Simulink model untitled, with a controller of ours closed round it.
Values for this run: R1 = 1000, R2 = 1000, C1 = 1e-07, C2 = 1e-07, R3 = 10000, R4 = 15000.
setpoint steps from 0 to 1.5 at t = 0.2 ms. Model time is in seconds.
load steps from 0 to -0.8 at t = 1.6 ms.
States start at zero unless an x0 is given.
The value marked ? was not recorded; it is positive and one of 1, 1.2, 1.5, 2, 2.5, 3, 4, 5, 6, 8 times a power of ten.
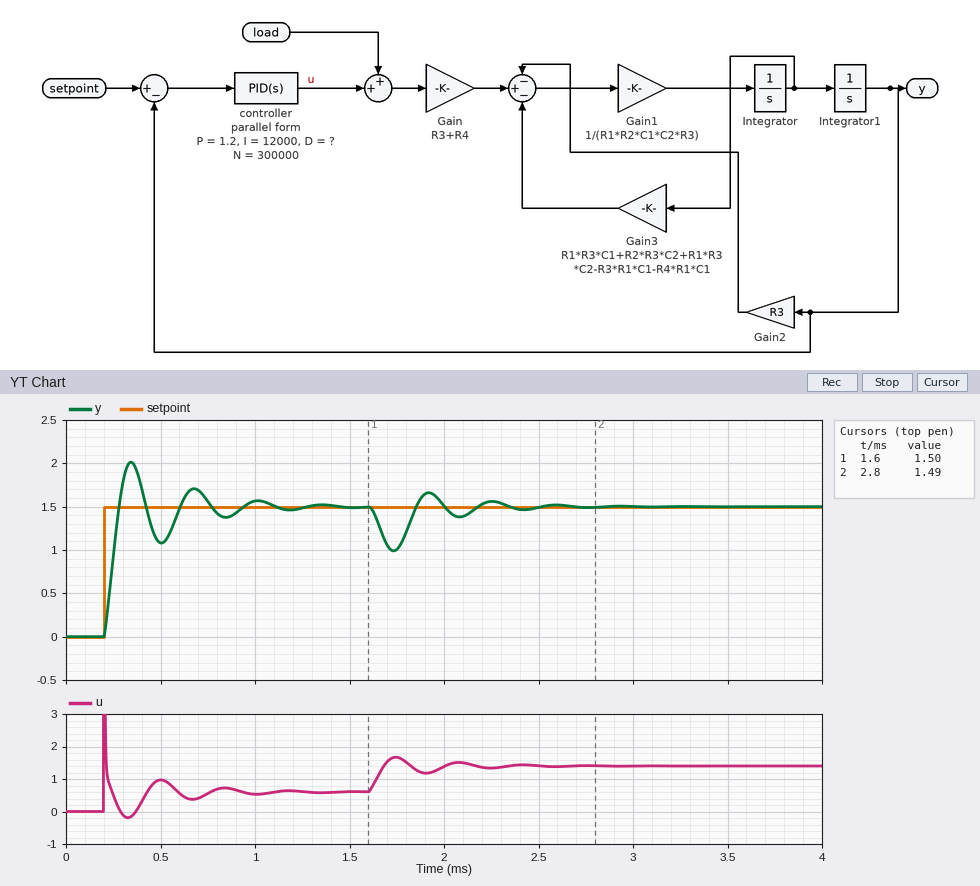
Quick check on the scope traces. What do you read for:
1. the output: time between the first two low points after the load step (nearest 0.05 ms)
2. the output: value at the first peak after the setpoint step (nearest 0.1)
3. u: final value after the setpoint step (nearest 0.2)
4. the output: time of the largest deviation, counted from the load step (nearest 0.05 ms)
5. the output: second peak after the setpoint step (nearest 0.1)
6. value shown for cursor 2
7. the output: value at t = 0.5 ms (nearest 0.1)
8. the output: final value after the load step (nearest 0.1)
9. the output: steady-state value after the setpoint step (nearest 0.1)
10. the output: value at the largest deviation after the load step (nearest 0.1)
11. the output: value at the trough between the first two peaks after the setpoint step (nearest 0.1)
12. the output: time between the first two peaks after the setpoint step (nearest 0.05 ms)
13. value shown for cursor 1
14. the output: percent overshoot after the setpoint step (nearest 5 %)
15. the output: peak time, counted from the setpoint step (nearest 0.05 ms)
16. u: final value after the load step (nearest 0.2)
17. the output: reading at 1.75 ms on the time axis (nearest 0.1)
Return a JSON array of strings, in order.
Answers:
["0.35 ms", "2.0", "0.6", "0.15 ms", "1.7", "1.49", "1.1", "1.5", "1.5", "1.0", "1.1", "0.35 ms", "1.50", "35 %", "0.15 ms", "1.4", "1.0"]
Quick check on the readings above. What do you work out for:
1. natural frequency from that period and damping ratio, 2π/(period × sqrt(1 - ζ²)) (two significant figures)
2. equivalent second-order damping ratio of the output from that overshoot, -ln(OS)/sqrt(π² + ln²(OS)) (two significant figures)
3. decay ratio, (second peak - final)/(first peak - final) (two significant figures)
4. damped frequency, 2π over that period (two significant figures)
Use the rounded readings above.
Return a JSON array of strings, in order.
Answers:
["19 rad/ms", "0.32", "0.40", "18 rad/ms"]
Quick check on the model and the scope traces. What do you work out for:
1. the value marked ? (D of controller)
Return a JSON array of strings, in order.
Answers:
["4e-05"]
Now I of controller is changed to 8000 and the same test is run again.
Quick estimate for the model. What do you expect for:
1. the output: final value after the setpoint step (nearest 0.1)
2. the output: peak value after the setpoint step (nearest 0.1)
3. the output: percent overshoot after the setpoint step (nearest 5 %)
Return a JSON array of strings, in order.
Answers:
["1.5", "1.9", "25 %"]
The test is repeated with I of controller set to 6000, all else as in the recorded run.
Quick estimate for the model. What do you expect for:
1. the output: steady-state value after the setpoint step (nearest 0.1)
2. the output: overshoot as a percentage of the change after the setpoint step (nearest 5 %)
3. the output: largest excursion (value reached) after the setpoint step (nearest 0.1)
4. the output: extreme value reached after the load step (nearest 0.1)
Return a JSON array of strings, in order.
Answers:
["1.5", "20 %", "1.8", "0.9"]
